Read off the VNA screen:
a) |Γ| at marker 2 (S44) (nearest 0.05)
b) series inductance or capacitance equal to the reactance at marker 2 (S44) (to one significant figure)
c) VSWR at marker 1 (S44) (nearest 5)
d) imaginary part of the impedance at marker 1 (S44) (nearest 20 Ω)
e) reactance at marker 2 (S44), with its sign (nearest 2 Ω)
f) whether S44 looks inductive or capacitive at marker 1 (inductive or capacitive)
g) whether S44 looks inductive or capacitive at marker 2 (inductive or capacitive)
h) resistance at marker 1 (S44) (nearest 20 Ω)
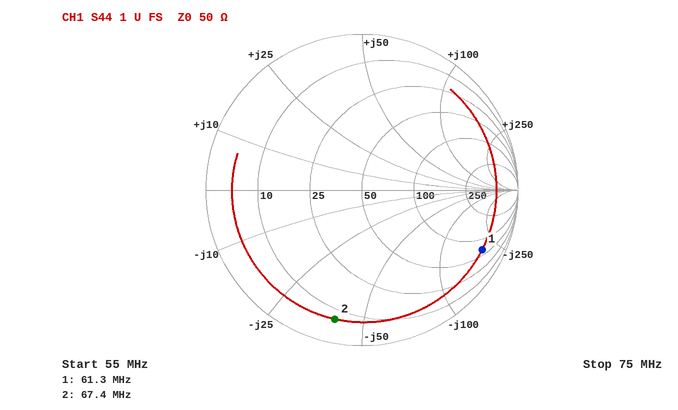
0.85
60 pF
15
-200 Ω
-40 Ω
capacitive
capacitive
60 Ω
